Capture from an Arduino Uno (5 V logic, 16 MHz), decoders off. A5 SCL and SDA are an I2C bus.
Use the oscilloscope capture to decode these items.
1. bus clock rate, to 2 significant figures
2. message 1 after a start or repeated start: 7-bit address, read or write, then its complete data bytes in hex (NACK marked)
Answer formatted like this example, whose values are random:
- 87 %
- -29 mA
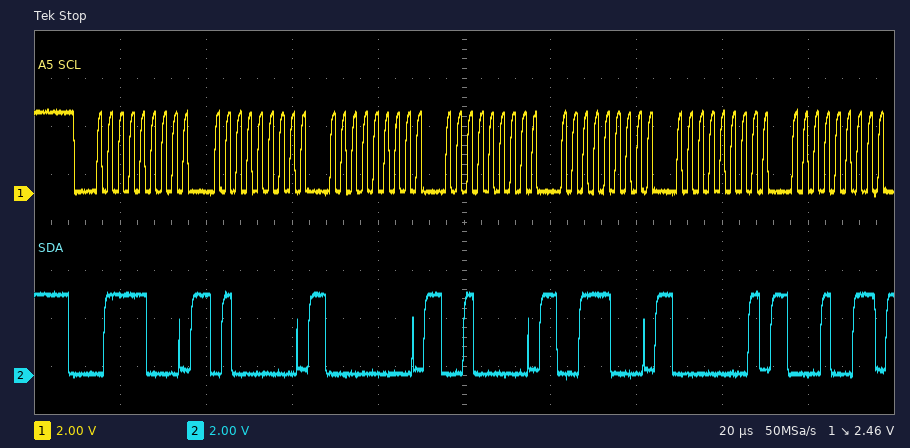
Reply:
- 400 kHz
- 0x3C write: 40 00 20 38 01 13
